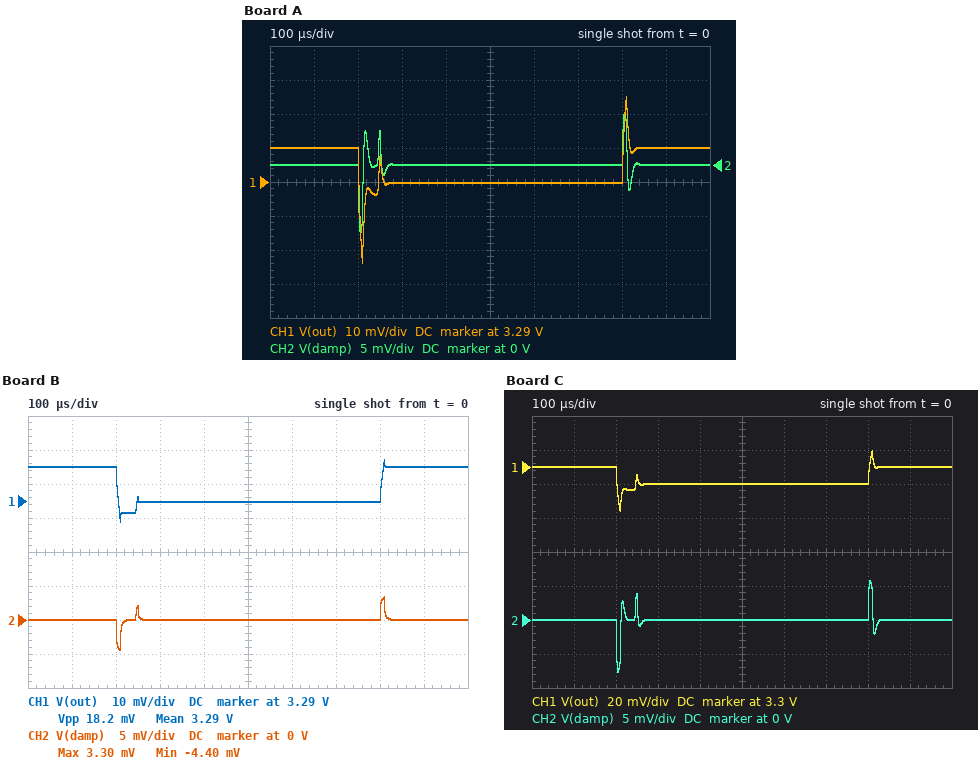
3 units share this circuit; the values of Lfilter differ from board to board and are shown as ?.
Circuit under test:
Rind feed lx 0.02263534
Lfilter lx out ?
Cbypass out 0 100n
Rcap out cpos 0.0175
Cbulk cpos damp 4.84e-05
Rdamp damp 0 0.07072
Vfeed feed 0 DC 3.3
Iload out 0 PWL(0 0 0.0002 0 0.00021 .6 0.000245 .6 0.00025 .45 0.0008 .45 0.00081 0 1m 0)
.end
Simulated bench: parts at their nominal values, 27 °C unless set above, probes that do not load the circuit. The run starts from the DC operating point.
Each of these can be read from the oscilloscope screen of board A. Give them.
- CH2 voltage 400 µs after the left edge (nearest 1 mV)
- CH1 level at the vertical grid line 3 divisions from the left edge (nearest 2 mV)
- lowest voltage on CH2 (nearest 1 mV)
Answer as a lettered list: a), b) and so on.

a) 0 V
b) 3.290 V
c) -10 mV
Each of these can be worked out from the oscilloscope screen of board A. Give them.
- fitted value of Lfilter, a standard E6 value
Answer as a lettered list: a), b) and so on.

a) 330 nH
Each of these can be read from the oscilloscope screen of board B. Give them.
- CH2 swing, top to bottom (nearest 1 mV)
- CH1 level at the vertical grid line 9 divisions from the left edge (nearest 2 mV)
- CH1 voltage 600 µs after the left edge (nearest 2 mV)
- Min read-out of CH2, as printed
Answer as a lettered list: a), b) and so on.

a) 8 mV
b) 3.300 V
c) 3.290 V
d) -4.40 mV
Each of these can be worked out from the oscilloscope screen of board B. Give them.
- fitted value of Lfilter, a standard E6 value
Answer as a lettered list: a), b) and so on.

a) 68 nH
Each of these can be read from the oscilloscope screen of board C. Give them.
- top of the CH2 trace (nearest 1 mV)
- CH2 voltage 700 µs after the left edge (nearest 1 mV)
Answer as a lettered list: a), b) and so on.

a) 6 mV
b) 0 V
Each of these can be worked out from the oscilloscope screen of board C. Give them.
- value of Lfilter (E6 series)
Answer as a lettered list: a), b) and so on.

a) 220 nH
